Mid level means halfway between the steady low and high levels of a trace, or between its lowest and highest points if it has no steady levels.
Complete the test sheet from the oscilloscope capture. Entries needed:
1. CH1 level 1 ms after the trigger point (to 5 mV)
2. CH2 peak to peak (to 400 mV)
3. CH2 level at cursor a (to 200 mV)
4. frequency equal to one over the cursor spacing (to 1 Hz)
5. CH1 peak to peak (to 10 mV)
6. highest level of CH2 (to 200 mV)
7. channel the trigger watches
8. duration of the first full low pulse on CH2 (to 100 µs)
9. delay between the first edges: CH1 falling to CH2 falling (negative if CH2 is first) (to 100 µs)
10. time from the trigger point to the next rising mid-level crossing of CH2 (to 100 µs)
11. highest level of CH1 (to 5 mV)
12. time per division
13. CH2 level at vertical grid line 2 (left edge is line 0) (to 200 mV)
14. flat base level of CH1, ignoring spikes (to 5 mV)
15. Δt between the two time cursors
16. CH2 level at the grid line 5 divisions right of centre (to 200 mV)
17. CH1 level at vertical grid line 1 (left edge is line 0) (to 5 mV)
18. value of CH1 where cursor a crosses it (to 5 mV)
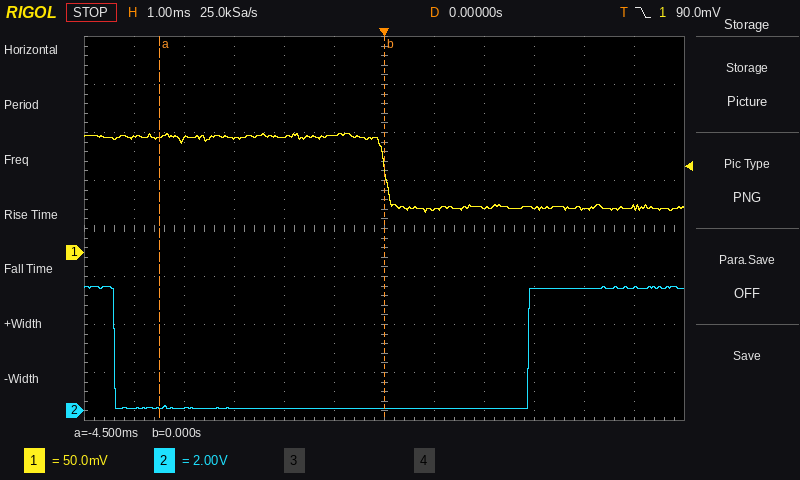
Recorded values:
45 mV
5.2 V
200 mV
222 Hz
80 mV
5.2 V
CH1
8.3 ms
-5.4 ms
2.9 ms
125 mV
1 ms
200 mV
45 mV
4.5 ms
5.2 V
120 mV
120 mV
